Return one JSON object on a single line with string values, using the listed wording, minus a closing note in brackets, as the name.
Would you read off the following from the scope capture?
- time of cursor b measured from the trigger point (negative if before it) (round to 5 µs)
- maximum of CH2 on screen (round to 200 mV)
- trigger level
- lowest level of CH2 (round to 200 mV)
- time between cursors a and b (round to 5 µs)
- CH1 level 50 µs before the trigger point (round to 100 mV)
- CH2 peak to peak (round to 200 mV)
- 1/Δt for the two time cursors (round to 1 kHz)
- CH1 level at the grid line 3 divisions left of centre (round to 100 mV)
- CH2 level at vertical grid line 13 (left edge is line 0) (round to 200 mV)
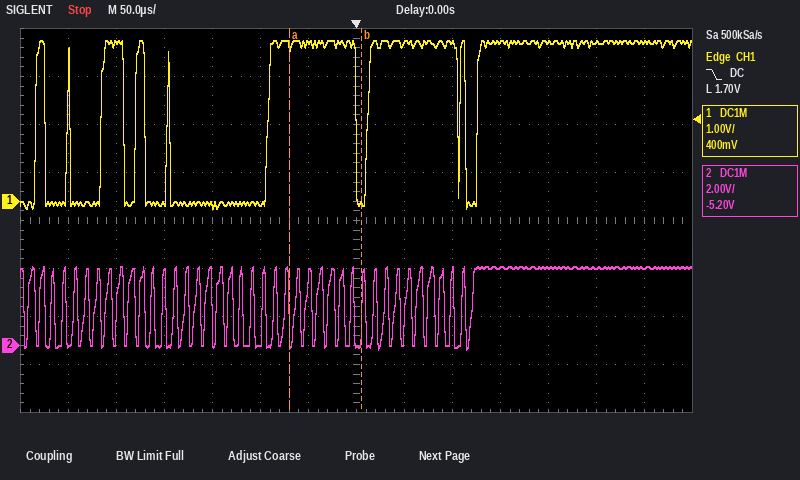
{"time of cursor b measured from the trigger point (negative if before it)": "+5 µs", "maximum of CH2 on screen": "3.2 V", "trigger level": "1.70 V", "lowest level of CH2": "-200 mV", "time between cursors a and b": "75 µs", "CH1 level 50 µs before the trigger point": "3.3 V", "CH2 peak to peak": "3.4 V", "1/Δt for the two time cursors": "13 kHz", "CH1 level at the grid line 3 divisions left of centre": "-100 mV", "CH2 level at vertical grid line 13 (left edge is line 0)": "3.2 V"}
